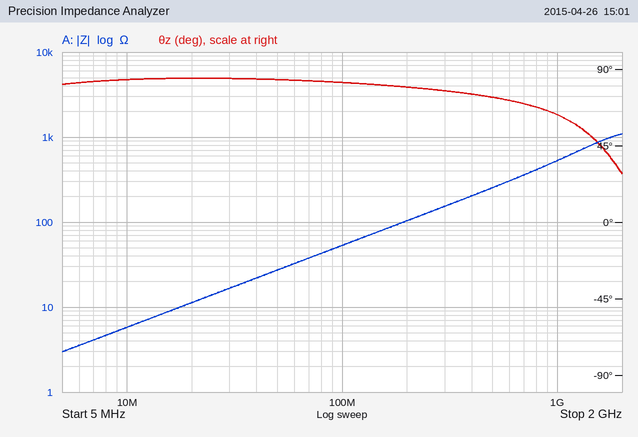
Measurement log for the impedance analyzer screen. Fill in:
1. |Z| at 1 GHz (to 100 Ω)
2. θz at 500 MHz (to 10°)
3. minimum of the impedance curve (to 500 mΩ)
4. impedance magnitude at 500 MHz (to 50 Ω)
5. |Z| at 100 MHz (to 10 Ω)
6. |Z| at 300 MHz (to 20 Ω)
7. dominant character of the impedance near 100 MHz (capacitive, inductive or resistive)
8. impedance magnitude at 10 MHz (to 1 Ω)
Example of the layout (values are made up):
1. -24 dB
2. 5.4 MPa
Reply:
1. 500 Ω
2. 70°
3. 3.0 Ω
4. 250 Ω
5. 50 Ω
6. 160 Ω
7. inductive
8. 6 Ω
